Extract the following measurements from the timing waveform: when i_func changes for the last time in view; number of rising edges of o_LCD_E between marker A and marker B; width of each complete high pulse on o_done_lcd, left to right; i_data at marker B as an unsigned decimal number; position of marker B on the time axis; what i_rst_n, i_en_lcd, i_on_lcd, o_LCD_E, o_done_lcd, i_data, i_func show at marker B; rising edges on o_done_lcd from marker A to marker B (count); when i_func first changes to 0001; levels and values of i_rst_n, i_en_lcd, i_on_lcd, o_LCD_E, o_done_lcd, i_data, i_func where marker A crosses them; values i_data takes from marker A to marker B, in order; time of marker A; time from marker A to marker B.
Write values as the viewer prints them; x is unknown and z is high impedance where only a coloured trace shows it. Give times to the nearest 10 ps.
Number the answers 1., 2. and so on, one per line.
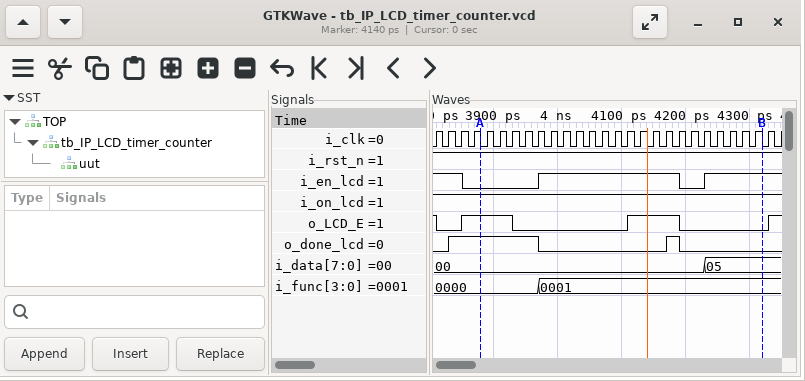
1. 3970 ps
2. 1
3. 140 ps, 20 ps
4. 5
5. 4320 ps
6. i_rst_n=1, i_en_lcd=1, i_on_lcd=1, o_LCD_E=0, o_done_lcd=0, i_data=05, i_func=0001
7. 1
8. 3970 ps
9. i_rst_n=1, i_en_lcd=0, i_on_lcd=1, o_LCD_E=1, o_done_lcd=1, i_data=00, i_func=0000
10. 00, 05
11. 3880 ps
12. 440 ps
